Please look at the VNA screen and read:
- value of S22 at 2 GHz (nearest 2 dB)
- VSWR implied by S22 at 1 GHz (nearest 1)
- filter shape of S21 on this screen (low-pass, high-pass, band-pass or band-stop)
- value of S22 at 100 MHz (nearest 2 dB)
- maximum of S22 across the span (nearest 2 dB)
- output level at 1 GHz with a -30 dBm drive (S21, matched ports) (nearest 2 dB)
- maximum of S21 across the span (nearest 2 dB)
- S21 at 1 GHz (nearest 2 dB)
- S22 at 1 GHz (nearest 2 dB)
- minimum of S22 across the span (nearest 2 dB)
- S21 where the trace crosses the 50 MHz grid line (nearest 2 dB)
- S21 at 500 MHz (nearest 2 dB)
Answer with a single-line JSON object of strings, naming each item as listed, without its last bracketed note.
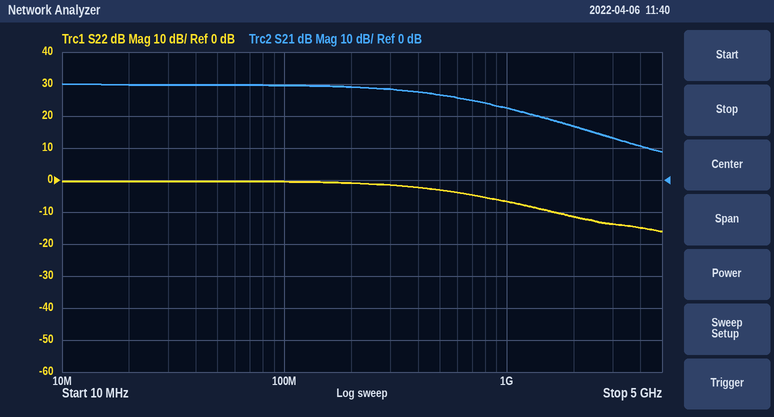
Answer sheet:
{"value of S22 at 2 GHz": "-12 dB", "VSWR implied by S22 at 1 GHz": "3", "filter shape of S21 on this screen": "low-pass", "value of S22 at 100 MHz": "0 dB", "maximum of S22 across the span": "0 dB", "output level at 1 GHz with a -30 dBm drive (S21, matched ports)": "-8 dBm", "maximum of S21 across the span": "30 dB", "S21 at 1 GHz": "22 dB", "S22 at 1 GHz": "-6 dB", "minimum of S22 across the span": "-16 dB", "S21 where the trace crosses the 50 MHz grid line": "30 dB", "S21 at 500 MHz": "26 dB"}
